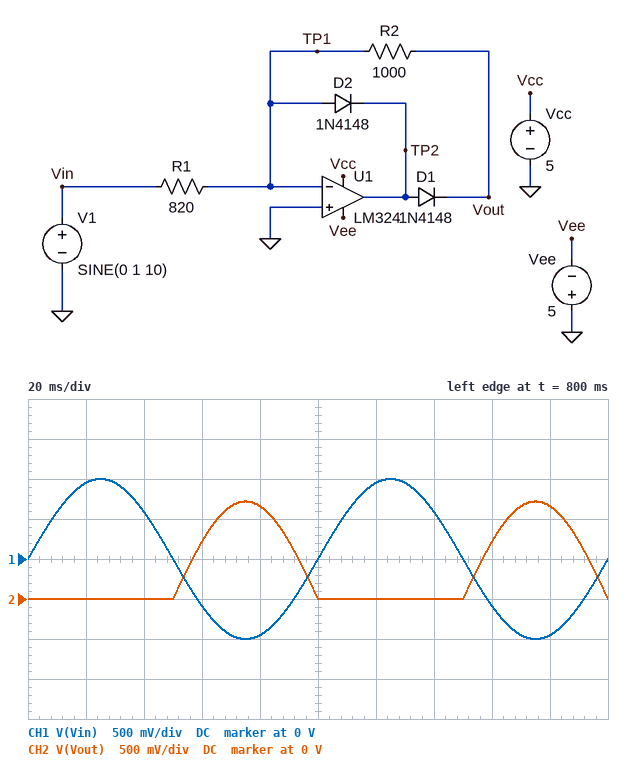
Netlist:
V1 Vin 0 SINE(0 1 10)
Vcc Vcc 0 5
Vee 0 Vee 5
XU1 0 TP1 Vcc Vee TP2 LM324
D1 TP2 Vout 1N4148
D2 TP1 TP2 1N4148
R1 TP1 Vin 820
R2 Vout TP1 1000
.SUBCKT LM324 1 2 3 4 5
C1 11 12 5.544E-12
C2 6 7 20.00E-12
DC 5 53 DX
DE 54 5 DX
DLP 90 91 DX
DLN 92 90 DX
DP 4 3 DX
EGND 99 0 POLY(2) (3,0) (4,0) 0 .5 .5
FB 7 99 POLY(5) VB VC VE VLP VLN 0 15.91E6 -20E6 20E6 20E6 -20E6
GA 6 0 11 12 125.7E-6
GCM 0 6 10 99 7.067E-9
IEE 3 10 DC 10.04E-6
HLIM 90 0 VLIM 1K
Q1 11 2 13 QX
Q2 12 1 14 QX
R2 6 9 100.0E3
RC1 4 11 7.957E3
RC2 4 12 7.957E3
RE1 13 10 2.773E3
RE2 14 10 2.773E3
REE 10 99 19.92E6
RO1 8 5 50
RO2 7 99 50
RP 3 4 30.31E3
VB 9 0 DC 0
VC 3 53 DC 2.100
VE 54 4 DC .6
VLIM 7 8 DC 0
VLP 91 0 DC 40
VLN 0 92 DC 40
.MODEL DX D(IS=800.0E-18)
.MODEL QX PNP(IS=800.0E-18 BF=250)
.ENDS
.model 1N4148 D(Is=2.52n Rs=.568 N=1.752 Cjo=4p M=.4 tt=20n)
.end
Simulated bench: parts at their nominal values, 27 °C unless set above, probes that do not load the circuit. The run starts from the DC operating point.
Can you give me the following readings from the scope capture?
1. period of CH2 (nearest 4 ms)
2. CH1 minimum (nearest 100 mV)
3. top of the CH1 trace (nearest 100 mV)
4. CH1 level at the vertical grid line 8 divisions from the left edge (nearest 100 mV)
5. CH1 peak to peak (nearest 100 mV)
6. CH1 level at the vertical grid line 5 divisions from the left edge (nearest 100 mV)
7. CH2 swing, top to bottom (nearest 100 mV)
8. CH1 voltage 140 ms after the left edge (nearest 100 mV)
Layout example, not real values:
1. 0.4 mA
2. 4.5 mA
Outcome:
1. 100 ms
2. -1.0 V
3. 1.0 V
4. -600 mV
5. 2.0 V
6. 0 V
7. 1.2 V
8. 600 mV
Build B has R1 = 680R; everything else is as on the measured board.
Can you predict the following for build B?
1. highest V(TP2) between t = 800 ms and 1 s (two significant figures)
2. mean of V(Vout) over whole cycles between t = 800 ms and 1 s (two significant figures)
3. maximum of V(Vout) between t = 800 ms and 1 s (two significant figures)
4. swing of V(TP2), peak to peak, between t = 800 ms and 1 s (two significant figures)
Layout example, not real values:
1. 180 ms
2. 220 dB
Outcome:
1. 2.1 V
2. 470 mV
3. 1.5 V
4. 2.7 V
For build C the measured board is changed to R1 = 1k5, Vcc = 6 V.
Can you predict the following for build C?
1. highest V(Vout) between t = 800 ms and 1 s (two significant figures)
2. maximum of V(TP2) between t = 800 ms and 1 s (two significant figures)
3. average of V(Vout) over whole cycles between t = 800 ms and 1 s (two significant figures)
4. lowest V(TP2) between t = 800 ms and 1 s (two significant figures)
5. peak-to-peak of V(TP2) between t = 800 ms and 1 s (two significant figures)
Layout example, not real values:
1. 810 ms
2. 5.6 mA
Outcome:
1. 670 mV
2. 1.2 V
3. 210 mV
4. -570 mV
5. 1.8 V
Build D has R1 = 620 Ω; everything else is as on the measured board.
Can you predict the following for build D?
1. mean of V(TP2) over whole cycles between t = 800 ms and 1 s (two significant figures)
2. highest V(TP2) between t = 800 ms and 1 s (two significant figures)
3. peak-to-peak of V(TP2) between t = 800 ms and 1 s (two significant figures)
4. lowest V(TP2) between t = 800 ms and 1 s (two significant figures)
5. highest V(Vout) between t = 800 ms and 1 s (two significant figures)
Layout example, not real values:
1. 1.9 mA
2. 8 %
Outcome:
1. 510 mV
2. 2.2 V
3. 2.8 V
4. -610 mV
5. 1.6 V
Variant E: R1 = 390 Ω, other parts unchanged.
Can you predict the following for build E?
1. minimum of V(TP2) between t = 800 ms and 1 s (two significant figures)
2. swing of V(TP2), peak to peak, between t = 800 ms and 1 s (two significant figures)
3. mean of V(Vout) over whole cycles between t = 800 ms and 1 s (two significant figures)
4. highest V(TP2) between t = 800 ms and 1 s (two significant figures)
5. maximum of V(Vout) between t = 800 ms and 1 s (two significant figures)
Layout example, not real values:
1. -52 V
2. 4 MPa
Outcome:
1. -630 mV
2. 3.8 V
3. 820 mV
4. 3.2 V
5. 2.6 V
